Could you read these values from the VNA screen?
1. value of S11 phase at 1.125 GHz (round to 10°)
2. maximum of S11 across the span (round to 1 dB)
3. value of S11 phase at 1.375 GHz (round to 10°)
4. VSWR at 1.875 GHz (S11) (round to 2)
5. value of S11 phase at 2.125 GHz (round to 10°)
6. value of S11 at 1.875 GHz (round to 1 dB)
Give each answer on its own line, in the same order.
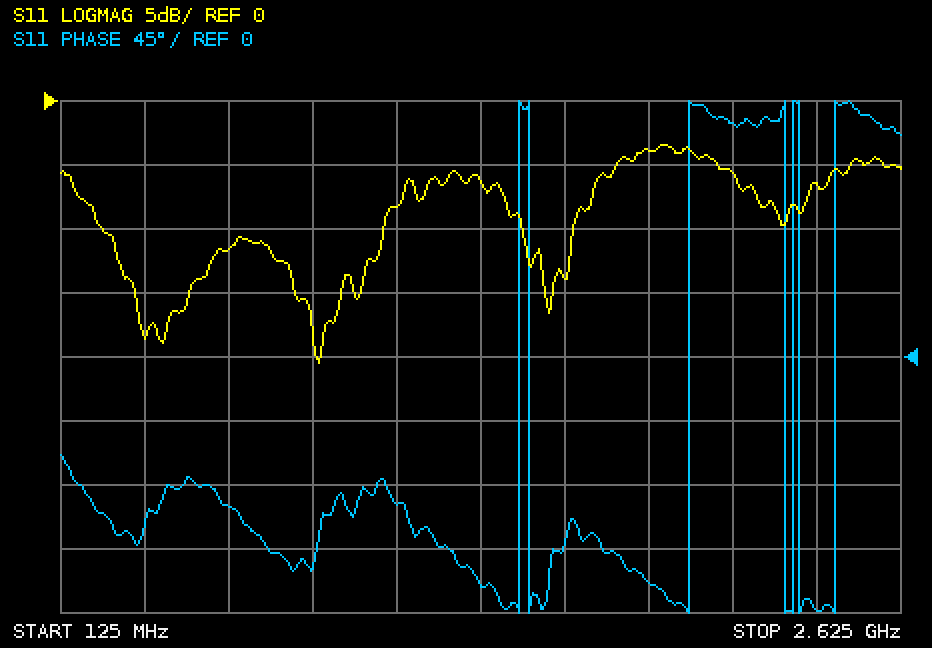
-100°
-3 dB
-160°
4
160°
-4 dB
